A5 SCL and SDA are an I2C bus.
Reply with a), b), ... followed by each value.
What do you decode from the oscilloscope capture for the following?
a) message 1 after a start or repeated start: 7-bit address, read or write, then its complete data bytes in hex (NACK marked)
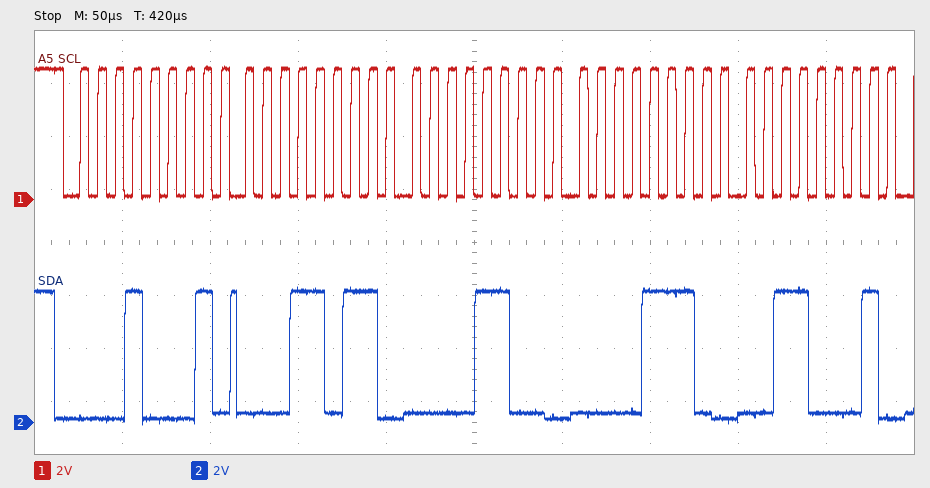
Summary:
a) 0x08 read: 1B 0C 0E 31
